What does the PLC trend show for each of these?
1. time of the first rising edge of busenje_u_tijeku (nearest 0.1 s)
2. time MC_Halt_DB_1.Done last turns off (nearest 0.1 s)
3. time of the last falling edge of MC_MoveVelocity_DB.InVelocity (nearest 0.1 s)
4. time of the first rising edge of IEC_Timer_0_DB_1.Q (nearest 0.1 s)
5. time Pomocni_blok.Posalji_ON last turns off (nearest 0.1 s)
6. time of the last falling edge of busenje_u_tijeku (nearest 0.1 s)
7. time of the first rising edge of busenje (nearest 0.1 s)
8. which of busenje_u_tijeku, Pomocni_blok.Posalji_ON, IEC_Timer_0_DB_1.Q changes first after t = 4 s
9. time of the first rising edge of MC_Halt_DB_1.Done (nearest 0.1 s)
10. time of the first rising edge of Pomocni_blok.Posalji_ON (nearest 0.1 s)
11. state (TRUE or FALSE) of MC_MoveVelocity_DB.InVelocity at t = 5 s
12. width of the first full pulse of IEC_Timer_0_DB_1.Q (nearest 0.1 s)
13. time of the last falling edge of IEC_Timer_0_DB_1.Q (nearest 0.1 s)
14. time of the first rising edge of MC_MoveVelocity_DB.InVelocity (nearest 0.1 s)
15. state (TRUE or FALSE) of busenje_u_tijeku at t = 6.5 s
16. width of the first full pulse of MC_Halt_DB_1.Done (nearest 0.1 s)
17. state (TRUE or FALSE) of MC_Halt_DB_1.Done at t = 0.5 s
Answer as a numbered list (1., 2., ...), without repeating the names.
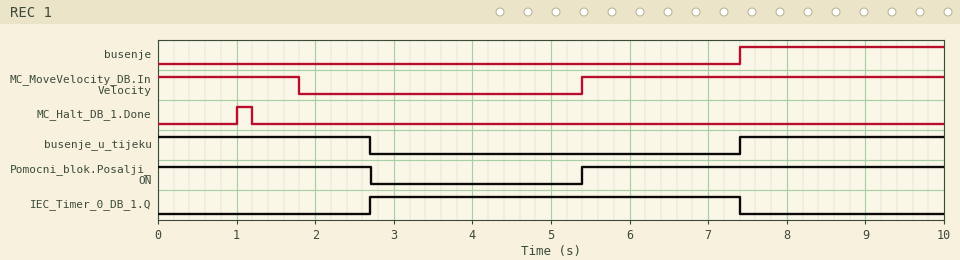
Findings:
1. 7.4 s
2. 1.2 s
3. 1.8 s
4. 2.7 s
5. 2.7 s
6. 2.7 s
7. 7.4 s
8. Pomocni_blok.Posalji_ON
9. 1.0 s
10. 5.4 s
11. FALSE
12. 4.7 s
13. 7.4 s
14. 5.4 s
15. FALSE
16. 0.2 s
17. FALSE
